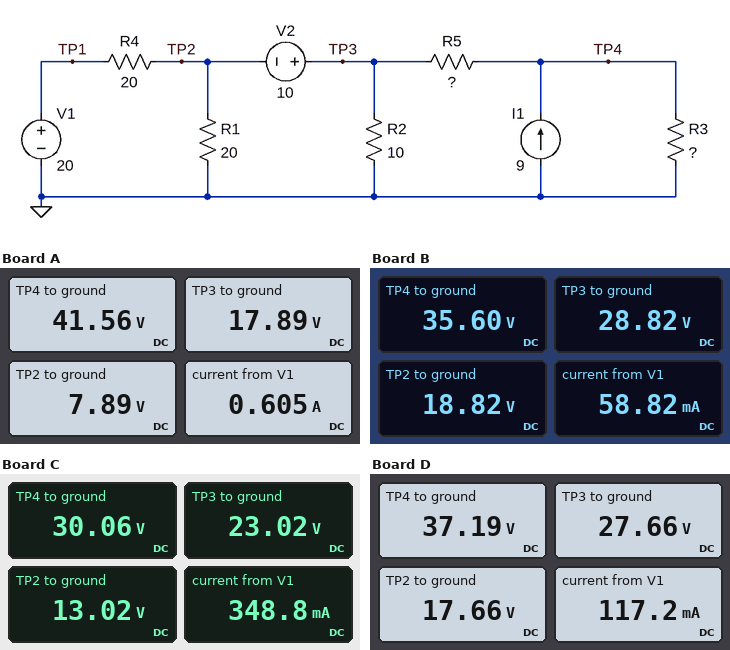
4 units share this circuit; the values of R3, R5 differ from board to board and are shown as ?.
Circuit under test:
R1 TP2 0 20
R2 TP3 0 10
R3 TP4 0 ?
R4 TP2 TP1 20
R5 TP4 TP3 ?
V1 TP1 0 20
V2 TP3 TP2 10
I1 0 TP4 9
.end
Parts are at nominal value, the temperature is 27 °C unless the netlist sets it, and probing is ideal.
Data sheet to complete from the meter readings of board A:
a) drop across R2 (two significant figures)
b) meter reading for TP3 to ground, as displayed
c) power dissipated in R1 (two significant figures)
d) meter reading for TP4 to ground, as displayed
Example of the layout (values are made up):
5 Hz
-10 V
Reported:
18 V
17.89 V
3.1 W
41.56 V
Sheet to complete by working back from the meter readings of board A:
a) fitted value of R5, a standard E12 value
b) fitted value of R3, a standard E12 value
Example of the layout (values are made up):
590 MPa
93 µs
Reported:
15 Ω
5.6 Ω
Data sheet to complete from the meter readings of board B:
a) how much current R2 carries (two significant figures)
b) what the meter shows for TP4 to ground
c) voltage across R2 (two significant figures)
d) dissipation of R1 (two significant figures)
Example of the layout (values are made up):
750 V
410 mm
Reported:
2.9 A
35.60 V
29 V
18 W
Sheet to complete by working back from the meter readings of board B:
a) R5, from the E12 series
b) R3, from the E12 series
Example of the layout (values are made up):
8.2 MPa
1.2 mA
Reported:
1.8 Ω
6.8 Ω
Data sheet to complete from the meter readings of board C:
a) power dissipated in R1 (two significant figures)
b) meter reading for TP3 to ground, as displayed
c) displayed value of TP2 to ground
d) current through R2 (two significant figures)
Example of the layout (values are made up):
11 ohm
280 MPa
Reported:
8.5 W
23.02 V
13.02 V
2.3 A
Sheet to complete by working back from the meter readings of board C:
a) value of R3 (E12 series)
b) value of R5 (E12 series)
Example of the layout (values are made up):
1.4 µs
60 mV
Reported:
4.7 Ω
2.7 Ω
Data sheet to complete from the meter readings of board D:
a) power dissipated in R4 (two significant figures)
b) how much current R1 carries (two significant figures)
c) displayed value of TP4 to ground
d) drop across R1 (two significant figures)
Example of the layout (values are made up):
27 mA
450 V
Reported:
270 mW
880 mA
37.19 V
18 V
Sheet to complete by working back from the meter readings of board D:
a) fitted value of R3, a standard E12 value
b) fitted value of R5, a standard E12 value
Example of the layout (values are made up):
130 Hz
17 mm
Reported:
6.8 Ω
2.7 Ω
